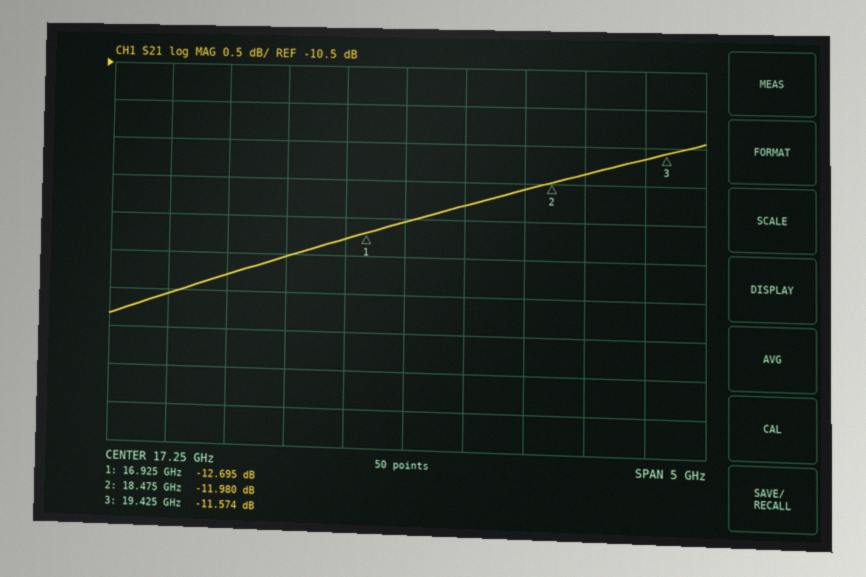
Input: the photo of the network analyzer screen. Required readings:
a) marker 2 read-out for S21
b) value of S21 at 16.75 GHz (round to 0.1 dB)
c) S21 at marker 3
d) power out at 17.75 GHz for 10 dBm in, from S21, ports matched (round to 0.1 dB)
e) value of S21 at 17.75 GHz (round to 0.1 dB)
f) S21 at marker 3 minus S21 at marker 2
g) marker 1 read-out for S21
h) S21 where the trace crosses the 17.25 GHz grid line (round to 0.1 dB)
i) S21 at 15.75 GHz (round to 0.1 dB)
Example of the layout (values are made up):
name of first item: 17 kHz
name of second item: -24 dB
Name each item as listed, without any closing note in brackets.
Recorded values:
marker 2 read-out for S21: -11.980 dB
value of S21 at 16.75 GHz: -12.8 dB
S21 at marker 3: -11.574 dB
power out at 17.75 GHz for 10 dBm in, from S21, ports matched: -2.3 dBm
value of S21 at 17.75 GHz: -12.3 dB
S21 at marker 3 minus S21 at marker 2: 0.406 dB
marker 1 read-out for S21: -12.695 dB
S21 where the trace crosses the 17.25 GHz grid line: -12.5 dB
S21 at 15.75 GHz: -13.3 dB
